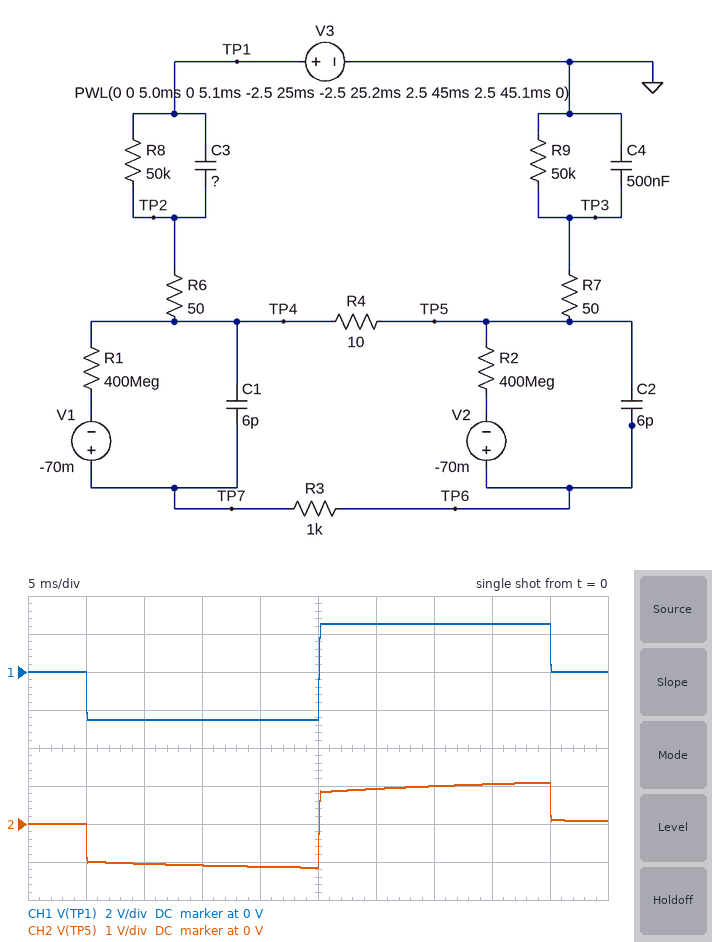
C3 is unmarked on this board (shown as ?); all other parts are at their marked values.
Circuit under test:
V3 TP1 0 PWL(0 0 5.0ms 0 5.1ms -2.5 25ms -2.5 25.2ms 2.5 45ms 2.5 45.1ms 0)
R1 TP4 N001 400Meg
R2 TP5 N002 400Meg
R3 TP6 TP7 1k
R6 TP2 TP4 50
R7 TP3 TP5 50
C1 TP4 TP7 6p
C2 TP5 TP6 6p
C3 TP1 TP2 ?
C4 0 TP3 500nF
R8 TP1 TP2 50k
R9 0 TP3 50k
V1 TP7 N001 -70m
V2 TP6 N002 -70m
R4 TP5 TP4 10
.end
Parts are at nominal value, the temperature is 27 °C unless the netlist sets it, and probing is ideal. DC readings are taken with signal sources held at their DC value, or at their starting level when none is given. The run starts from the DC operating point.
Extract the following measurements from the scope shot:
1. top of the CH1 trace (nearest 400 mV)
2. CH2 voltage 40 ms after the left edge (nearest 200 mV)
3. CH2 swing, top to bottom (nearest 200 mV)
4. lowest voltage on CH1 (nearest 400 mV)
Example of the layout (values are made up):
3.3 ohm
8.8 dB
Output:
2.4 V
1.0 V
2.2 V
-2.4 V
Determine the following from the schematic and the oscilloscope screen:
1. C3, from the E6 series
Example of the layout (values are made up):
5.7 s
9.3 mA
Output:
330 nF
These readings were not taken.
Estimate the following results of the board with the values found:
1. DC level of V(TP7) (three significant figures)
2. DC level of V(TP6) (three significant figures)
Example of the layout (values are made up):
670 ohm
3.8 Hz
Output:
-70.0 mV
-70.0 mV
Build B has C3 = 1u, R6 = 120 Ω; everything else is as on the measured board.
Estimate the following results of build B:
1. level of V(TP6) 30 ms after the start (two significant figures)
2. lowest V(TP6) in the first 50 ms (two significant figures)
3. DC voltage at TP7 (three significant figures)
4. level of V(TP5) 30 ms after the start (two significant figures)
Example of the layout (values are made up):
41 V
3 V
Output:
1.7 V
-1.7 V
-70.0 mV
1.8 V
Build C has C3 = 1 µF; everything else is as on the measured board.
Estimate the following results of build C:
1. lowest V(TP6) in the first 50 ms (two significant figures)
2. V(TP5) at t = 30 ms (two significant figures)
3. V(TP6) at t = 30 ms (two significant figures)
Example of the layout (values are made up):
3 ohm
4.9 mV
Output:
-1.7 V
1.8 V
1.7 V
